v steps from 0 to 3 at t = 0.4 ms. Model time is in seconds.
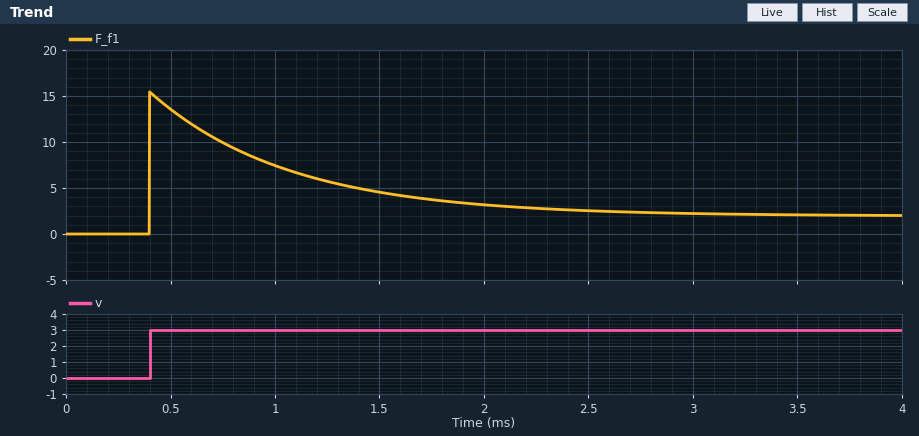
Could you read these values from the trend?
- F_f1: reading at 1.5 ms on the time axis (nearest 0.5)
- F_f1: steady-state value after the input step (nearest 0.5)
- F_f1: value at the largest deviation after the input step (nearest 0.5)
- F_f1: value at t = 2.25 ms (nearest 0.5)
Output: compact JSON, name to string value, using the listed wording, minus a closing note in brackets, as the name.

{"F_f1: reading at 1.5 ms on the time axis": "4.5", "F_f1: steady-state value after the input step": "2.0", "F_f1: value at the largest deviation after the input step": "15.5", "F_f1: value at t = 2.25 ms": "3.0"}
